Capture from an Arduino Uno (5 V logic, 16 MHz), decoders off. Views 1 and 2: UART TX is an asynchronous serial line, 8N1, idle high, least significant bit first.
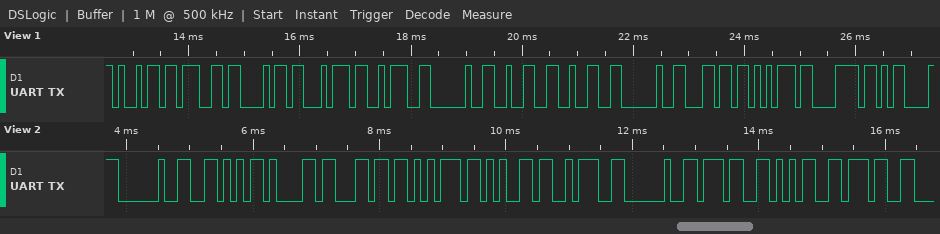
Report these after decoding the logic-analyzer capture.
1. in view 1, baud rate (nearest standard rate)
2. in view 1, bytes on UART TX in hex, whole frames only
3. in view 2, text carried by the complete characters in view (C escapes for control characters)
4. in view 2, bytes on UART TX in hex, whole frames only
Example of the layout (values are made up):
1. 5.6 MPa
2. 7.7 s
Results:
1. 9600 baud
2. 69 67 68 74 3A 20 32 32 20 6C 75 78 0D
3. " Value: 757"
4. 20 56 61 6C 75 65 3A 20 37 35 37
